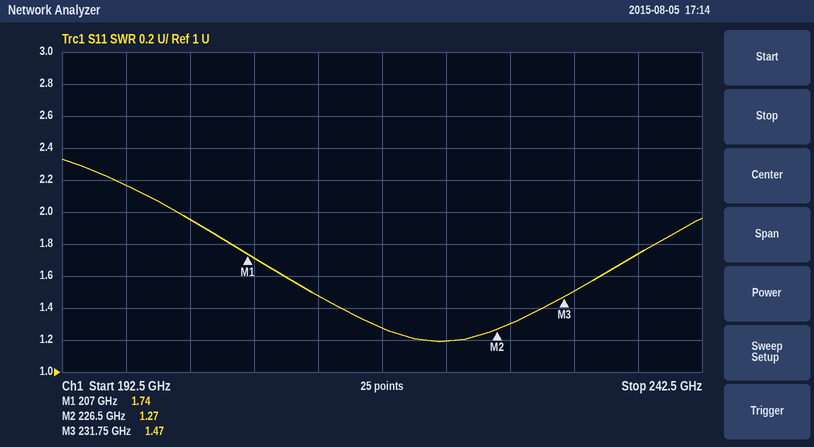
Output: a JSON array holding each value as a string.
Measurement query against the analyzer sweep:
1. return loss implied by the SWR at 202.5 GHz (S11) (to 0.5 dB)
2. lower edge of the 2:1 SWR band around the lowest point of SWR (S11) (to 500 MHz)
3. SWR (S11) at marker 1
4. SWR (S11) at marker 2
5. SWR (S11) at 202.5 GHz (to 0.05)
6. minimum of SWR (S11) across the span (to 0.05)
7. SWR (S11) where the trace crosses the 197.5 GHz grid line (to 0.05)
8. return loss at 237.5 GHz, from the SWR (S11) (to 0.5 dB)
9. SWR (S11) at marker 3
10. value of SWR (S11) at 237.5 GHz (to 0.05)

["10.0 dB", "201.5 GHz", "1.74", "1.27", "1.95", "1.20", "2.15", "11.5 dB", "1.47", "1.75"]
